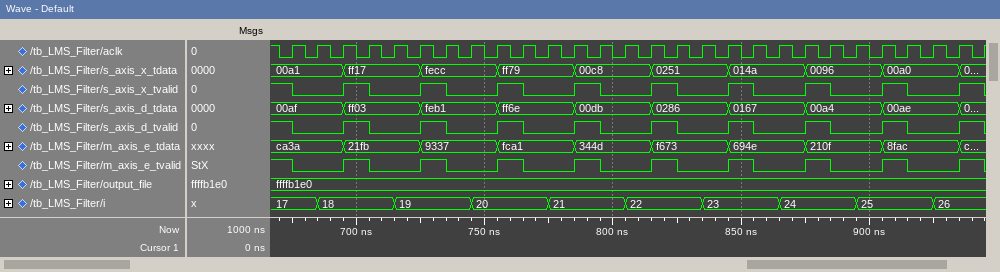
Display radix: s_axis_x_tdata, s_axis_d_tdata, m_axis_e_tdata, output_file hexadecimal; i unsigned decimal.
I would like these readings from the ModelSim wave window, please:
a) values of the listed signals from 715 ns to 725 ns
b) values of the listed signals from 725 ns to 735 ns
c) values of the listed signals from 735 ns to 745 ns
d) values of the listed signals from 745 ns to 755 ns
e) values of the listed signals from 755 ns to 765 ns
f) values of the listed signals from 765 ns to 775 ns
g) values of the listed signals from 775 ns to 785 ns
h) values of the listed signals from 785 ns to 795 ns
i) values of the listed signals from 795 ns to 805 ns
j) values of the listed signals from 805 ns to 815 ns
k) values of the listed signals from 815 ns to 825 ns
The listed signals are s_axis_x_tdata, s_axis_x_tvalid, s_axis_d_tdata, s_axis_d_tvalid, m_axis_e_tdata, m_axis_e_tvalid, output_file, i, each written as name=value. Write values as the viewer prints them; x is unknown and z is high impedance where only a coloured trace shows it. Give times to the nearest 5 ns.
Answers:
s_axis_x_tdata=ff17, s_axis_x_tvalid=0, s_axis_d_tdata=ff03, s_axis_d_tvalid=0, m_axis_e_tdata=21fb, m_axis_e_tvalid=0, output_file=ffffb1e0, i=19
s_axis_x_tdata=fecc, s_axis_x_tvalid=1, s_axis_d_tdata=feb1, s_axis_d_tvalid=1, m_axis_e_tdata=9337, m_axis_e_tvalid=1, output_file=ffffb1e0, i=19
s_axis_x_tdata=fecc, s_axis_x_tvalid=0, s_axis_d_tdata=feb1, s_axis_d_tvalid=0, m_axis_e_tdata=9337, m_axis_e_tvalid=0, output_file=ffffb1e0, i=19
s_axis_x_tdata=fecc, s_axis_x_tvalid=0, s_axis_d_tdata=feb1, s_axis_d_tvalid=0, m_axis_e_tdata=9337, m_axis_e_tvalid=0, output_file=ffffb1e0, i=20
s_axis_x_tdata=ff79, s_axis_x_tvalid=1, s_axis_d_tdata=ff6e, s_axis_d_tvalid=1, m_axis_e_tdata=fca1, m_axis_e_tvalid=1, output_file=ffffb1e0, i=20
s_axis_x_tdata=ff79, s_axis_x_tvalid=0, s_axis_d_tdata=ff6e, s_axis_d_tvalid=0, m_axis_e_tdata=fca1, m_axis_e_tvalid=0, output_file=ffffb1e0, i=20
s_axis_x_tdata=ff79, s_axis_x_tvalid=0, s_axis_d_tdata=ff6e, s_axis_d_tvalid=0, m_axis_e_tdata=fca1, m_axis_e_tvalid=0, output_file=ffffb1e0, i=21
s_axis_x_tdata=00c8, s_axis_x_tvalid=1, s_axis_d_tdata=00db, s_axis_d_tvalid=1, m_axis_e_tdata=344d, m_axis_e_tvalid=1, output_file=ffffb1e0, i=21
s_axis_x_tdata=00c8, s_axis_x_tvalid=0, s_axis_d_tdata=00db, s_axis_d_tvalid=0, m_axis_e_tdata=344d, m_axis_e_tvalid=0, output_file=ffffb1e0, i=21
s_axis_x_tdata=00c8, s_axis_x_tvalid=0, s_axis_d_tdata=00db, s_axis_d_tvalid=0, m_axis_e_tdata=344d, m_axis_e_tvalid=0, output_file=ffffb1e0, i=22
s_axis_x_tdata=0251, s_axis_x_tvalid=1, s_axis_d_tdata=0286, s_axis_d_tvalid=1, m_axis_e_tdata=f673, m_axis_e_tvalid=1, output_file=ffffb1e0, i=22
